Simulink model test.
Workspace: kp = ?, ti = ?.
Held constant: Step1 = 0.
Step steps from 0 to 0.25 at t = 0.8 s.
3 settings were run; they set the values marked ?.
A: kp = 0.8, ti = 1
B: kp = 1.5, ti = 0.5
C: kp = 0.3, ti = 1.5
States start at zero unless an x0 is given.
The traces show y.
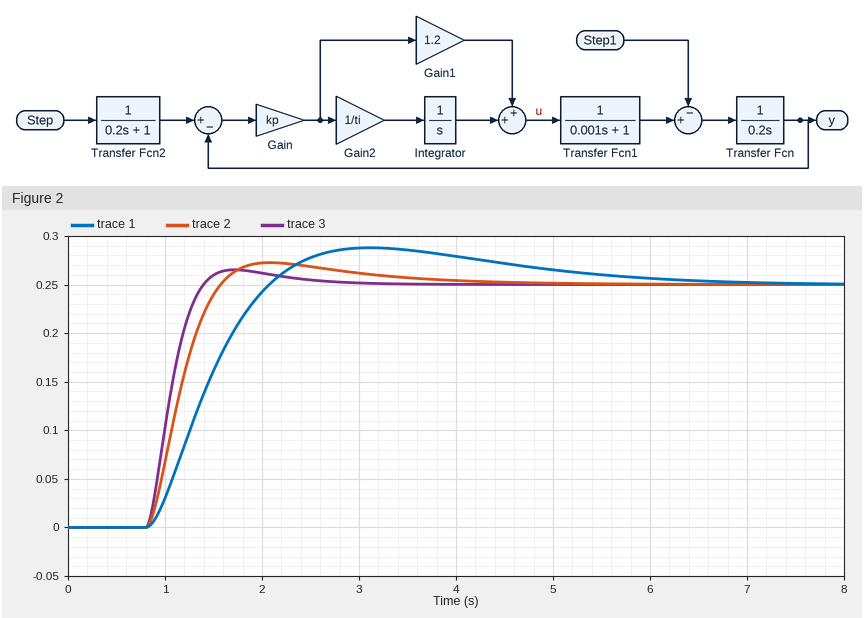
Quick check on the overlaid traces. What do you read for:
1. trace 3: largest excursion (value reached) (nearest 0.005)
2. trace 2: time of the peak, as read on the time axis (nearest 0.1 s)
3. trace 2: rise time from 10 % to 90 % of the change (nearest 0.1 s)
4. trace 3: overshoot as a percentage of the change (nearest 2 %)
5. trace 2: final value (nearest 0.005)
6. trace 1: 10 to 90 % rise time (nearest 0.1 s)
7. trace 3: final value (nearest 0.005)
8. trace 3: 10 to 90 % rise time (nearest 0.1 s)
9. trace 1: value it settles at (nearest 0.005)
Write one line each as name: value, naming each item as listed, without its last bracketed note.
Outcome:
trace 3: largest excursion (value reached): 0.265
trace 2: time of the peak, as read on the time axis: 2.1 s
trace 2: rise time from 10 % to 90 % of the change: 0.5 s
trace 3: overshoot as a percentage of the change: 6 %
trace 2: final value: 0.250
trace 1: 10 to 90 % rise time: 0.9 s
trace 3: final value: 0.250
trace 3: 10 to 90 % rise time: 0.4 s
trace 1: value it settles at: 0.250
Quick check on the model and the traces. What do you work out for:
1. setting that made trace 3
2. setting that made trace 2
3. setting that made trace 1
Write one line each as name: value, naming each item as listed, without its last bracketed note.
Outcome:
setting that made trace 3: B
setting that made trace 2: A
setting that made trace 1: C
